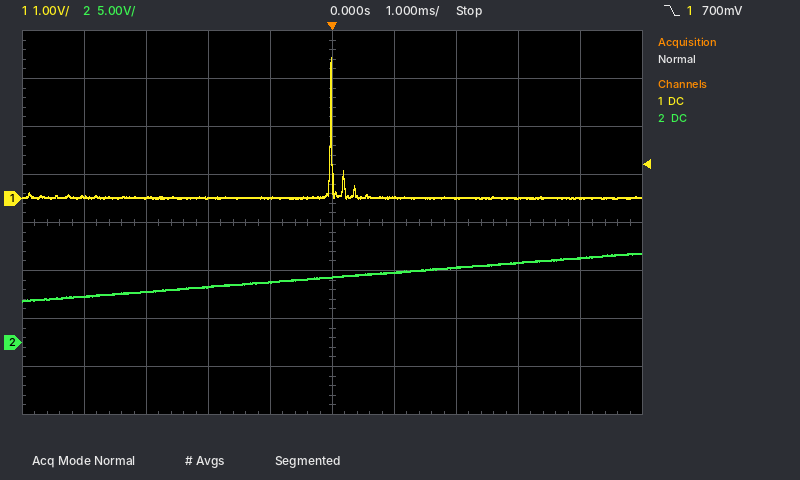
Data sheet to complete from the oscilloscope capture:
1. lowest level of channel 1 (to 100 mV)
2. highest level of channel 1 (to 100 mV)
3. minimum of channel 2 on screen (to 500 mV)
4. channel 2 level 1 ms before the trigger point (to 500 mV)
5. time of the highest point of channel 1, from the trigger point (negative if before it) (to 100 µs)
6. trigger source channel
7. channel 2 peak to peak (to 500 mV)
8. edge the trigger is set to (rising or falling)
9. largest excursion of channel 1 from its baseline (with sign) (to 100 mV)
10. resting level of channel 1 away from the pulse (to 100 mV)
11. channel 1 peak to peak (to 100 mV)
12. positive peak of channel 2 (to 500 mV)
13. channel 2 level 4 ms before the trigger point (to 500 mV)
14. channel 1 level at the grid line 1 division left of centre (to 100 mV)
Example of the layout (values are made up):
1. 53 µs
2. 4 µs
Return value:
1. 0.0 V
2. 2.9 V
3. 4.5 V
4. 6.5 V
5. 0.0 ms
6. channel 1
7. 5.0 V
8. falling
9. +2.9 V
10. 0.0 V
11. 2.9 V
12. 9.5 V
13. 5.0 V
14. 0.0 V
